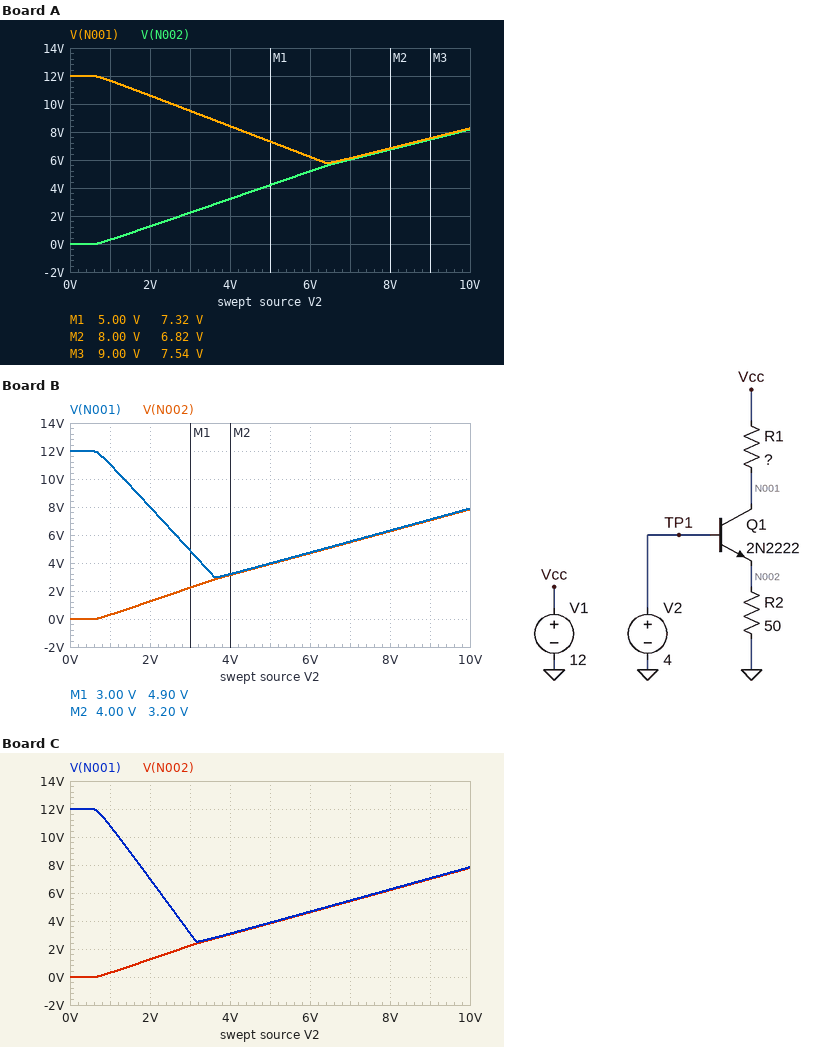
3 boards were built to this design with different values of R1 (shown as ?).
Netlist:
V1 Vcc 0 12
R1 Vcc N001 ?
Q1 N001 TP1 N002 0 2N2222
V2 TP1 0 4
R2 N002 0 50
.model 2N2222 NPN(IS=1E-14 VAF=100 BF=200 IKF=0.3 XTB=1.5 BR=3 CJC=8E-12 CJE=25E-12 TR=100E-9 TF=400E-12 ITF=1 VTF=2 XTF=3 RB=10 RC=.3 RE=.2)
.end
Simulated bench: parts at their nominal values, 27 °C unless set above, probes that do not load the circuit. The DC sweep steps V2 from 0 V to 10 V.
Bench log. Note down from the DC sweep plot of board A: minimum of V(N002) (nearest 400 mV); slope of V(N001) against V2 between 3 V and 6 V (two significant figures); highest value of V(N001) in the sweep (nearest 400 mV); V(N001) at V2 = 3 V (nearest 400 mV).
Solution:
0 V
-1.1 V/V
12.0 V
9.6 V
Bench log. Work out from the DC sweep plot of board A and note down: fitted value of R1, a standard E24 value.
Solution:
56 Ω
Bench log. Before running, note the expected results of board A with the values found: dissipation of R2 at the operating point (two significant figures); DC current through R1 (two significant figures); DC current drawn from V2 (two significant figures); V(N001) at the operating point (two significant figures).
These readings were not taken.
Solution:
210 mW
64 mA
370 µA
8.4 V
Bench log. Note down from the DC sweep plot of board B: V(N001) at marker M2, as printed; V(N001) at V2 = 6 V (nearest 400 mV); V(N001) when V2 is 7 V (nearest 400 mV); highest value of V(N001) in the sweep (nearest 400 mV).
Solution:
3.20 V
4.8 V
5.6 V
12.0 V
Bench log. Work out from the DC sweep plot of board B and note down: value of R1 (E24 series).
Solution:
160 Ω
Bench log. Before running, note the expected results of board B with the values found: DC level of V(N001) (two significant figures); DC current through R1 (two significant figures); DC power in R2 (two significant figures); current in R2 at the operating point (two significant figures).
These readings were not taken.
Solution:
3.2 V
55 mA
200 mW
63 mA
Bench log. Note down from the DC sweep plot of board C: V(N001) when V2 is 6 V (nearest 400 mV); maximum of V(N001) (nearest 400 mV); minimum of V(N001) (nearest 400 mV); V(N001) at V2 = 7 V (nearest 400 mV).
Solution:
4.8 V
12.0 V
2.4 V
5.6 V
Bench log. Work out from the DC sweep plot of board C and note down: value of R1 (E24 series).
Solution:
200 Ω
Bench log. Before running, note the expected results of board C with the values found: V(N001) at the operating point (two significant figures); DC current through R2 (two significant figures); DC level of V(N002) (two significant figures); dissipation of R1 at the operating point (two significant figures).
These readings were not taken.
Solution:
3.1 V
61 mA
3.0 V
400 mW
